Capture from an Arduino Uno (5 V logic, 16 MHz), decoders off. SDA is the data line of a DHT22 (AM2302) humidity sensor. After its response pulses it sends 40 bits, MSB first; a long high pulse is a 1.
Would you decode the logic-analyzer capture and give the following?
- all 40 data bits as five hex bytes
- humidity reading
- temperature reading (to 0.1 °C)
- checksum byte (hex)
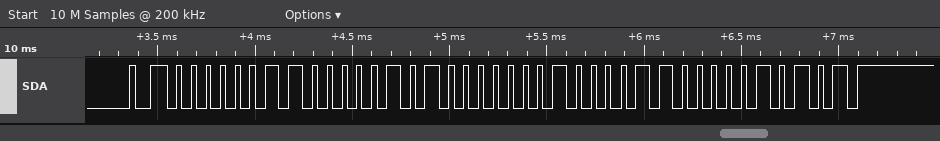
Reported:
03 05 01 0C 15
77.3 %
26.8 °C
0x15
